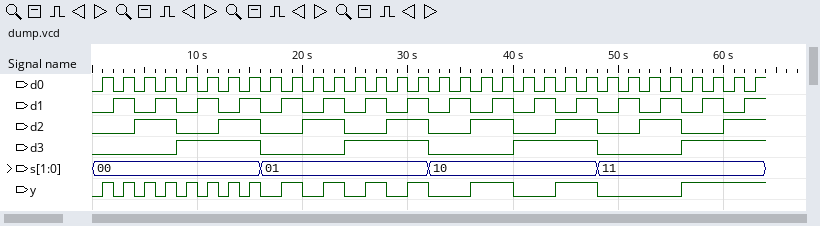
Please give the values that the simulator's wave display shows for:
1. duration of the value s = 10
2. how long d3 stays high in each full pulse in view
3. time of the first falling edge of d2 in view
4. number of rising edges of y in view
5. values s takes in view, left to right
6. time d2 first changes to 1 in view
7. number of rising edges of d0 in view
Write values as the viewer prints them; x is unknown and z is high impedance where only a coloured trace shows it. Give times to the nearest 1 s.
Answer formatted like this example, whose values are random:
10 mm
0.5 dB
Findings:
16 s
8 s, 8 s, 8 s
8 s
15
00, 01, 10, 11
4 s
32
